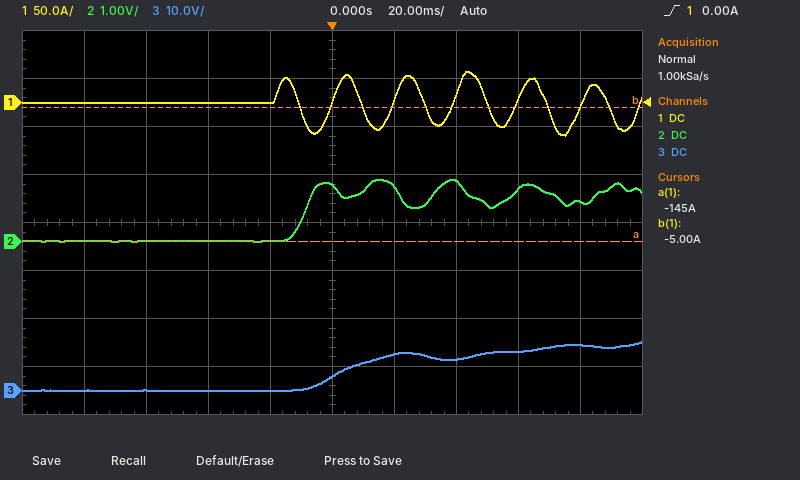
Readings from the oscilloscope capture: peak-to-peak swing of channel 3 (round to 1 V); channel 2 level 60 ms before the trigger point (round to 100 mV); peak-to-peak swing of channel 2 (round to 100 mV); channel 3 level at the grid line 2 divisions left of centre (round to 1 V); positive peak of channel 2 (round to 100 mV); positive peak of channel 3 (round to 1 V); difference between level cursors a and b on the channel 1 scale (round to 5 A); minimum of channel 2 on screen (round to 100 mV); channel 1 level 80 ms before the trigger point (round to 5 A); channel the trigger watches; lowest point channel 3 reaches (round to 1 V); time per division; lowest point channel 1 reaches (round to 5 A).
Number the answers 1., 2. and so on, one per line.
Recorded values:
1. 10 V
2. 0.0 V
3. 1.3 V
4. 0 V
5. 1.3 V
6. 10 V
7. 140 A
8. 0.0 V
9. 0 A
10. channel 1
11. 0 V
12. 20 ms
13. -35 A
